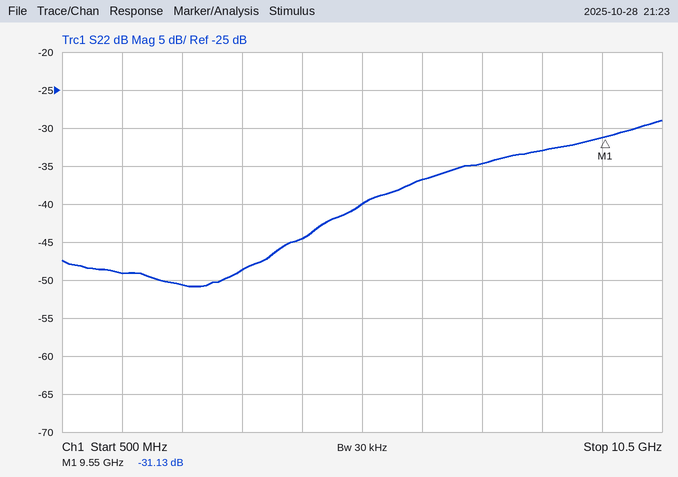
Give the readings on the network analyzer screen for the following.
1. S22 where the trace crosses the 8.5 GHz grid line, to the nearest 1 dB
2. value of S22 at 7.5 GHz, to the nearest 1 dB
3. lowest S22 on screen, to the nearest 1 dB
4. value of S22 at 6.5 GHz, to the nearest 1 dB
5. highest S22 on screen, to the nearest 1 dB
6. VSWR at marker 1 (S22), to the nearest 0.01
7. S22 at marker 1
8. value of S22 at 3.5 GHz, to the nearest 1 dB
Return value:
-33 dB
-35 dB
-51 dB
-37 dB
-29 dB
1.06
-31.13 dB
-49 dB
